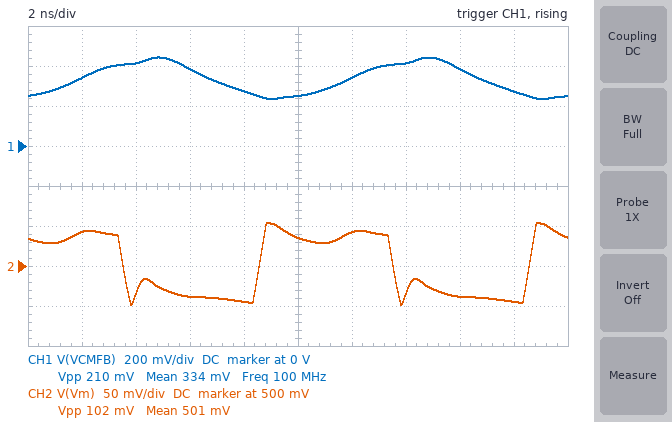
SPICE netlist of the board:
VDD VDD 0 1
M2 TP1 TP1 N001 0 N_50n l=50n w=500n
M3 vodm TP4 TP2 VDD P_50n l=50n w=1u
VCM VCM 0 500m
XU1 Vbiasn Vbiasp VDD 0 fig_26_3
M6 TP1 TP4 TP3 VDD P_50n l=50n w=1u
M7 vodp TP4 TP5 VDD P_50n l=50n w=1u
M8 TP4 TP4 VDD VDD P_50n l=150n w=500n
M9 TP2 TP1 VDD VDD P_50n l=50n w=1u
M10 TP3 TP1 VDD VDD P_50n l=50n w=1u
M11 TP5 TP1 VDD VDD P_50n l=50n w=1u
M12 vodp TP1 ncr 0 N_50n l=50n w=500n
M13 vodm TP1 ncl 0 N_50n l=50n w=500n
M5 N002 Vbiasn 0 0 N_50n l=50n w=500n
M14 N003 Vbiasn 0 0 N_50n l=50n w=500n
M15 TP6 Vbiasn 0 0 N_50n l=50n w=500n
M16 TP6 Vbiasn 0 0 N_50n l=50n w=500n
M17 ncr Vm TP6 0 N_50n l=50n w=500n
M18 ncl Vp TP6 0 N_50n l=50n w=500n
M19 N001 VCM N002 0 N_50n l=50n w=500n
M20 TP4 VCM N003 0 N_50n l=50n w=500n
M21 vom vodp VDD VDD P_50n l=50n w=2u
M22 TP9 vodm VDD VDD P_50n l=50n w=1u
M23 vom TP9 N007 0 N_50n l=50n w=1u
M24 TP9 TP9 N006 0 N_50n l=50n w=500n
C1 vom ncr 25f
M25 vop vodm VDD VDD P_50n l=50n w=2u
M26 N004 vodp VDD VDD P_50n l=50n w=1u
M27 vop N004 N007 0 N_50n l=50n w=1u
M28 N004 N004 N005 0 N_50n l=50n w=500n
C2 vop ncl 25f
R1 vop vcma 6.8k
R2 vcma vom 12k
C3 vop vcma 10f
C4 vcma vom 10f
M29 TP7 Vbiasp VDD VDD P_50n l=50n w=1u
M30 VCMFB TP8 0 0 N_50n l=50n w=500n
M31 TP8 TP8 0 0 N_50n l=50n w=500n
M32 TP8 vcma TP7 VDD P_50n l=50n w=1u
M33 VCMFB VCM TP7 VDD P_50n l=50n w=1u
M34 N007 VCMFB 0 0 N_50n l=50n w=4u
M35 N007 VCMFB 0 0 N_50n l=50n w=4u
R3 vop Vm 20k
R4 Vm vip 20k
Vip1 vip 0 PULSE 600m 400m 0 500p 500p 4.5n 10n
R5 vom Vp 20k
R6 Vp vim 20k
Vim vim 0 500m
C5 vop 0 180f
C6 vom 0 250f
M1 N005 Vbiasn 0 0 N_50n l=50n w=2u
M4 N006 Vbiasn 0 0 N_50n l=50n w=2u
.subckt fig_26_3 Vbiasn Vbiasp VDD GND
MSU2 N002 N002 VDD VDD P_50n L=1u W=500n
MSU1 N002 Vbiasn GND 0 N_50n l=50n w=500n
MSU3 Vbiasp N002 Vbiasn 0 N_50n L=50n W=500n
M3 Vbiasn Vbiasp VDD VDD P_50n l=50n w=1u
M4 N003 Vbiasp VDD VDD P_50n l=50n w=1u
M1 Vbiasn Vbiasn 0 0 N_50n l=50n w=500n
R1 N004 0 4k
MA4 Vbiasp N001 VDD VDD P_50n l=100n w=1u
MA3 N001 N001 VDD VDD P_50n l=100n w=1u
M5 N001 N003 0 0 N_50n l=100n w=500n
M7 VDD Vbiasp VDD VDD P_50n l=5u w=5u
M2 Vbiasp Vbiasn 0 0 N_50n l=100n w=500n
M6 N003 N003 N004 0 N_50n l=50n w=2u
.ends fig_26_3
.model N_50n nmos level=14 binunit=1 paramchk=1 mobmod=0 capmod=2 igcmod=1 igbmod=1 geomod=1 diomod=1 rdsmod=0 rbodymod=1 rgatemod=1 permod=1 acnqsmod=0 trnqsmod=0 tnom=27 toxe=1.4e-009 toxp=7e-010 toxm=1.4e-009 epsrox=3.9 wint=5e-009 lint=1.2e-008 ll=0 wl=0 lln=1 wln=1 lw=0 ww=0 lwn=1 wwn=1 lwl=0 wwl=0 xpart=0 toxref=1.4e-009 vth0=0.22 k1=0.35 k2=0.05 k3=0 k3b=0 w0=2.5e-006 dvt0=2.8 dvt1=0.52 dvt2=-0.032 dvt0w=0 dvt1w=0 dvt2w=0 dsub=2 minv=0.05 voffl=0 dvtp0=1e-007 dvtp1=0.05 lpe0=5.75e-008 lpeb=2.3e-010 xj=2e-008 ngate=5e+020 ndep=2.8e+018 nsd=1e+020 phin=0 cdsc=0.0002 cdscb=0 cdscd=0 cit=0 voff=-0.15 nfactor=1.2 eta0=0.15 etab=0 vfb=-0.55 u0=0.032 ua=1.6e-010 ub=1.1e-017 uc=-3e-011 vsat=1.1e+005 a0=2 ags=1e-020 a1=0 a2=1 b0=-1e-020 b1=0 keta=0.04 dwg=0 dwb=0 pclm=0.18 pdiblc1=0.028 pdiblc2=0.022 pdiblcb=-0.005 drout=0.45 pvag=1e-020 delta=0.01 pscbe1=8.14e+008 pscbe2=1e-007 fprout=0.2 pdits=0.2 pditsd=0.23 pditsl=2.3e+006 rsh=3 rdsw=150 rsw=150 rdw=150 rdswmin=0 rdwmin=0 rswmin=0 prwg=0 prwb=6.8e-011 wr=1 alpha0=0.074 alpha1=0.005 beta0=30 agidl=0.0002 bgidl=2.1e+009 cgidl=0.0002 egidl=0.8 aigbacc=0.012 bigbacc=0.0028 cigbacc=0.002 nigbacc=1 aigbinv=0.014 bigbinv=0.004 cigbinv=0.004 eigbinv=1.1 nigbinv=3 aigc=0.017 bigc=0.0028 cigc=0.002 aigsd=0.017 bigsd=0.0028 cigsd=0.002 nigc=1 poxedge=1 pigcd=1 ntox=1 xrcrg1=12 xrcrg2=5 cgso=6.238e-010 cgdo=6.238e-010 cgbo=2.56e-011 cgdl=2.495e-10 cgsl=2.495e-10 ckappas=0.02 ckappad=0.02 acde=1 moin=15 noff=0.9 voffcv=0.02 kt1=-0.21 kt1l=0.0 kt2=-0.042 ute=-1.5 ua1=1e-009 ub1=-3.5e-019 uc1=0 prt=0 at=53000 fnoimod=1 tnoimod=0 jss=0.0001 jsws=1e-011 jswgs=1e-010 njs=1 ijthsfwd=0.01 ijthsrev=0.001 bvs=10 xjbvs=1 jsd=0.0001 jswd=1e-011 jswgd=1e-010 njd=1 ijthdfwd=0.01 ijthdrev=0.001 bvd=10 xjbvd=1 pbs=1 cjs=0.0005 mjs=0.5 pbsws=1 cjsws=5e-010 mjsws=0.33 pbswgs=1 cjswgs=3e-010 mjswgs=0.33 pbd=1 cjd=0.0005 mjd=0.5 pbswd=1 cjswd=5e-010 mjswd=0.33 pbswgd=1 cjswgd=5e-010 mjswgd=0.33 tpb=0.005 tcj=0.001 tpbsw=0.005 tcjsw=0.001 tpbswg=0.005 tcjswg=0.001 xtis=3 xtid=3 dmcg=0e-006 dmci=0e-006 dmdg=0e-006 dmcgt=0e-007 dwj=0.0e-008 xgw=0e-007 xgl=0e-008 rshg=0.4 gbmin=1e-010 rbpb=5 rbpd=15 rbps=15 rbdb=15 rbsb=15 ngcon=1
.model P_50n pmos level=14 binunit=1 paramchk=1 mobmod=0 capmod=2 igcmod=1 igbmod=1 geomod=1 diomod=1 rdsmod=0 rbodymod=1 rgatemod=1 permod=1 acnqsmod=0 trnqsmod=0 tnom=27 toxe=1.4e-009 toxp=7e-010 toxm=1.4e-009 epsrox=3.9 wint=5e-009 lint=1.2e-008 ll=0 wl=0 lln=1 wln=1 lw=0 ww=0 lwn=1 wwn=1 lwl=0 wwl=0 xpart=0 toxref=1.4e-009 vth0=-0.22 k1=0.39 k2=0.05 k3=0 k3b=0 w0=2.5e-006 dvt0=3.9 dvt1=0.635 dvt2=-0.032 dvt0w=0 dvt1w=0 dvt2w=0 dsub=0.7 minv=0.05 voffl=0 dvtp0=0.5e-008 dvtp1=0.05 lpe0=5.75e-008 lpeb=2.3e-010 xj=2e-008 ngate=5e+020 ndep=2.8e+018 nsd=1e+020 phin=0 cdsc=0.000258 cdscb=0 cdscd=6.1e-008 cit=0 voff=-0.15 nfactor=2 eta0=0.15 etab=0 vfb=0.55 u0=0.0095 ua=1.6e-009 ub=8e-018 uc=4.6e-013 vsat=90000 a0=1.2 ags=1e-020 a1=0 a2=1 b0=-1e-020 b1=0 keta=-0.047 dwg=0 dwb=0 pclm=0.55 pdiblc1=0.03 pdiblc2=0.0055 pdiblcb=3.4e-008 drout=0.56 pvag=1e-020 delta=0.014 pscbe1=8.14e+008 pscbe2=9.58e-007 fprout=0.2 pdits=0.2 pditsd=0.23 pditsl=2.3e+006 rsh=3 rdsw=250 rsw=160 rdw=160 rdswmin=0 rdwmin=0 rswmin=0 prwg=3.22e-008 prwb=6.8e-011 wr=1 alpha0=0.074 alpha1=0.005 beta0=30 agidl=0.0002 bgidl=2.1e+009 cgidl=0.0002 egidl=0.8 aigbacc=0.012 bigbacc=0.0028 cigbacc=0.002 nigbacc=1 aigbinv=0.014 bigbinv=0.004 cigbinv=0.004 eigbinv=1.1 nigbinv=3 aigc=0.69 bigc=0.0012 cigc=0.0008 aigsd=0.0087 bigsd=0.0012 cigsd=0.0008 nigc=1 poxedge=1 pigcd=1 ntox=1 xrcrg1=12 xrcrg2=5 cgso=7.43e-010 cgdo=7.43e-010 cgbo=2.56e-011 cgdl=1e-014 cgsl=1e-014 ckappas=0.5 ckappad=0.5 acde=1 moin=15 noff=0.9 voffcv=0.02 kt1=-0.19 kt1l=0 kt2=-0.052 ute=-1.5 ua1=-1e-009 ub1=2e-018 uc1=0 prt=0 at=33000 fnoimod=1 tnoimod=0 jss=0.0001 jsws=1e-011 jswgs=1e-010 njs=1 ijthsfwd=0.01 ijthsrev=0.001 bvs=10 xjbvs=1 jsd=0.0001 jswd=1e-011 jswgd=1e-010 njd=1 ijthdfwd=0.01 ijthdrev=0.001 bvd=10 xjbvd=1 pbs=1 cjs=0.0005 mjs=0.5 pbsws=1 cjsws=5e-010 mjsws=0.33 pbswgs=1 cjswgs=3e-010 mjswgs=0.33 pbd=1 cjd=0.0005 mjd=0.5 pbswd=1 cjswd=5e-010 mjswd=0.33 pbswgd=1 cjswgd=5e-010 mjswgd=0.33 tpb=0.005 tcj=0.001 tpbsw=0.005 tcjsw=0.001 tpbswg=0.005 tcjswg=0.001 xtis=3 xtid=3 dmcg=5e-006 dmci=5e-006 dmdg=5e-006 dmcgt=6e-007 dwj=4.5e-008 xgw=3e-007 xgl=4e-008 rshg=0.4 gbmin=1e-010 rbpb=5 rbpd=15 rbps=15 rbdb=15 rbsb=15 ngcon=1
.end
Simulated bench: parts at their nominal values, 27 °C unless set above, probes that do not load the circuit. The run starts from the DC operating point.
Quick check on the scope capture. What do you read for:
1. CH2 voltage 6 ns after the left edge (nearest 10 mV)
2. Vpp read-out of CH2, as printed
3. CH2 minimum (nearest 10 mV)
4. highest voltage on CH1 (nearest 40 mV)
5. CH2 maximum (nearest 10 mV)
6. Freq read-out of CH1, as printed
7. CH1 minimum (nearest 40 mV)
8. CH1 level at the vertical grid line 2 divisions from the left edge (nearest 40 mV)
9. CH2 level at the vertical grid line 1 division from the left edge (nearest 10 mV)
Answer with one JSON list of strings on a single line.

["460 mV", "102 mV", "450 mV", "440 mV", "550 mV", "100 MHz", "240 mV", "400 mV", "540 mV"]
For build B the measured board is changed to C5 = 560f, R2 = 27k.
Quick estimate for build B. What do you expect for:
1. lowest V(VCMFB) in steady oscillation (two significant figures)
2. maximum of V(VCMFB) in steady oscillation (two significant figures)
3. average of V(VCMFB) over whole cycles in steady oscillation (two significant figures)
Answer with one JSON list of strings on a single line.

["260 mV", "470 mV", "340 mV"]
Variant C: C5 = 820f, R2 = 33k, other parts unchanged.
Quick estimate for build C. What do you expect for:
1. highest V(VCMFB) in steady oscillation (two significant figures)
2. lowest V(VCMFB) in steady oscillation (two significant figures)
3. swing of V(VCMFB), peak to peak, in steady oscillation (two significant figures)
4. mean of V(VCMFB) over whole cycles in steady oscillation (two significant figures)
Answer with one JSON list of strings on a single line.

["480 mV", "250 mV", "220 mV", "350 mV"]
